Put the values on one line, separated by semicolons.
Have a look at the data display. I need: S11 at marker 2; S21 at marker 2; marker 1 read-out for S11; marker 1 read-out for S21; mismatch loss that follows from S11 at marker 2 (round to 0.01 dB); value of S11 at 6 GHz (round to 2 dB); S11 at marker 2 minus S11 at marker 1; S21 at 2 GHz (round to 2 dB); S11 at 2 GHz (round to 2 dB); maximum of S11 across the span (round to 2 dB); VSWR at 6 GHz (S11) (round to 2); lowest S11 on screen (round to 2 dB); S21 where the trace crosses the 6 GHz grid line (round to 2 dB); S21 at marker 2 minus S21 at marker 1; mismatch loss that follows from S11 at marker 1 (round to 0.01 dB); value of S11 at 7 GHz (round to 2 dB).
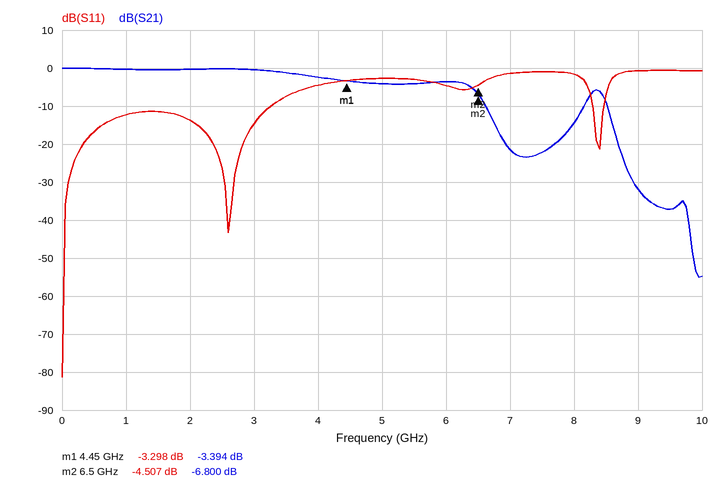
-4.507 dB; -6.800 dB; -3.298 dB; -3.394 dB; 1.90 dB; -4 dB; -1.209 dB; 0 dB; -14 dB; 0 dB; 4; -82 dB; -4 dB; -3.406 dB; 2.74 dB; -2 dB
